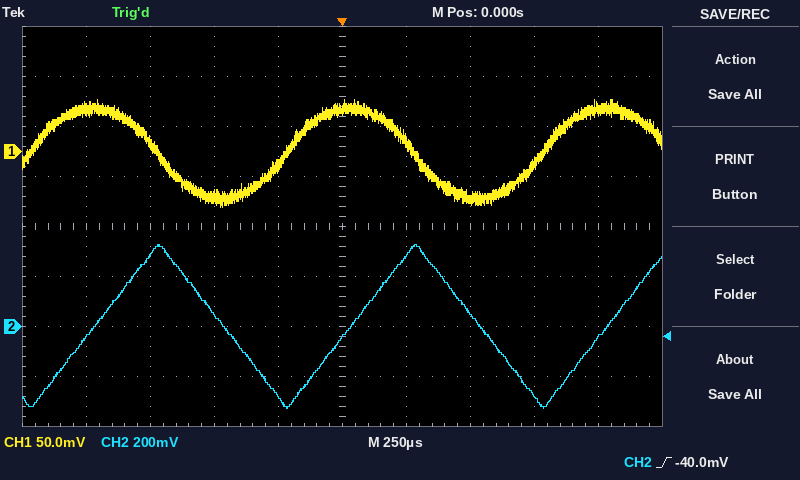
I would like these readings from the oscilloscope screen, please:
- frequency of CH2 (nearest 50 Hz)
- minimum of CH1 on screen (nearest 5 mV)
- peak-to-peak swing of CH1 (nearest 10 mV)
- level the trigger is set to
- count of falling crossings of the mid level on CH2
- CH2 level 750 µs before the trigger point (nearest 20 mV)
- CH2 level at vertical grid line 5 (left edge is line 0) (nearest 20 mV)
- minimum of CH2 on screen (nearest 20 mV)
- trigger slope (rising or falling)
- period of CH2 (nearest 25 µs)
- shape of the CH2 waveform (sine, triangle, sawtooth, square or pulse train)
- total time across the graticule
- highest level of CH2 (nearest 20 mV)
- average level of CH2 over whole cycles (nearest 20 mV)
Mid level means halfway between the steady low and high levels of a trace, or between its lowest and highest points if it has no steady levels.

1.00 kHz
-55 mV
110 mV
-40.0 mV
2
280 mV
-40 mV
-320 mV
rising
1.000 ms
triangle
2.5 ms
320 mV
0 mV
